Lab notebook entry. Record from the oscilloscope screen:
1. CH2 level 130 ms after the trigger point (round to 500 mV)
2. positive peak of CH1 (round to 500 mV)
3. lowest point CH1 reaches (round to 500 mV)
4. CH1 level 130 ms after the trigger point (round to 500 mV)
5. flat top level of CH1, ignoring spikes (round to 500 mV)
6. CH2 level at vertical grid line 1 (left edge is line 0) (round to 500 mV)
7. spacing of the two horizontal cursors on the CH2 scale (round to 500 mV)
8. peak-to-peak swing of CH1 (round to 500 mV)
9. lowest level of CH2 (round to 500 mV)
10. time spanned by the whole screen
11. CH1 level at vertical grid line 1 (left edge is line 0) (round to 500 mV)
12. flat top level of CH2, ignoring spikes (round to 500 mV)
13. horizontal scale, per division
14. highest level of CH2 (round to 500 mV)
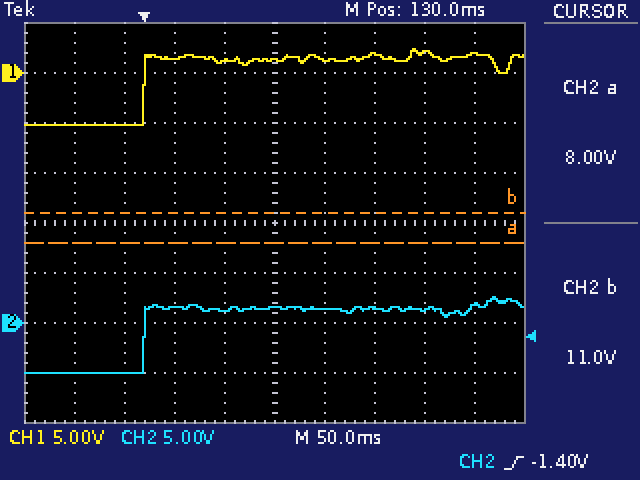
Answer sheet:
1.5 V
2.5 V
-5.0 V
1.5 V
1.5 V
-5.0 V
3.0 V
7.5 V
-5.0 V
500 ms
-5.0 V
1.5 V
50 ms
2.5 V
